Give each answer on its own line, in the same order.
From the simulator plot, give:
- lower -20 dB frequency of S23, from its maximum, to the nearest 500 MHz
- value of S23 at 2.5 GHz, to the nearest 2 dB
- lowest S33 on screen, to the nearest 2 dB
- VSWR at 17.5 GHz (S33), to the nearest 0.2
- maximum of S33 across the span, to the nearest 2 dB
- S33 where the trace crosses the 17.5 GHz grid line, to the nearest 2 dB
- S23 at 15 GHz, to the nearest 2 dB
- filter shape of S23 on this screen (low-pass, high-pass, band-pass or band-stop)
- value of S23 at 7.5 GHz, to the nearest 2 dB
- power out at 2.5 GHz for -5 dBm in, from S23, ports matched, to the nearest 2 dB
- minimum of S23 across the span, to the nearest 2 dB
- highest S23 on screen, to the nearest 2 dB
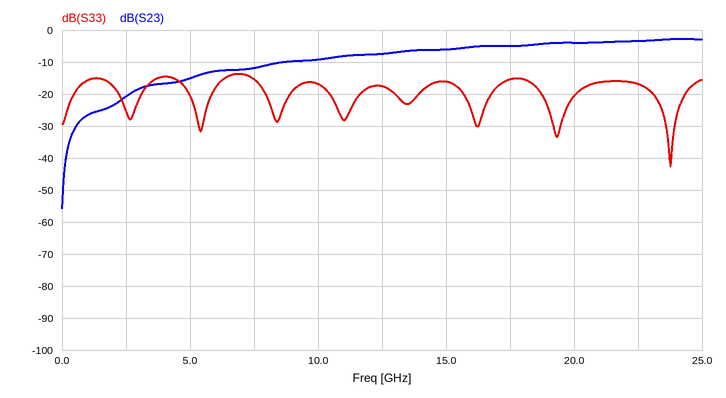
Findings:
2.0 GHz
-20 dB
-42 dB
1.4
-14 dB
-16 dB
-6 dB
high-pass
-12 dB
-26 dBm
-56 dB
-2 dB
